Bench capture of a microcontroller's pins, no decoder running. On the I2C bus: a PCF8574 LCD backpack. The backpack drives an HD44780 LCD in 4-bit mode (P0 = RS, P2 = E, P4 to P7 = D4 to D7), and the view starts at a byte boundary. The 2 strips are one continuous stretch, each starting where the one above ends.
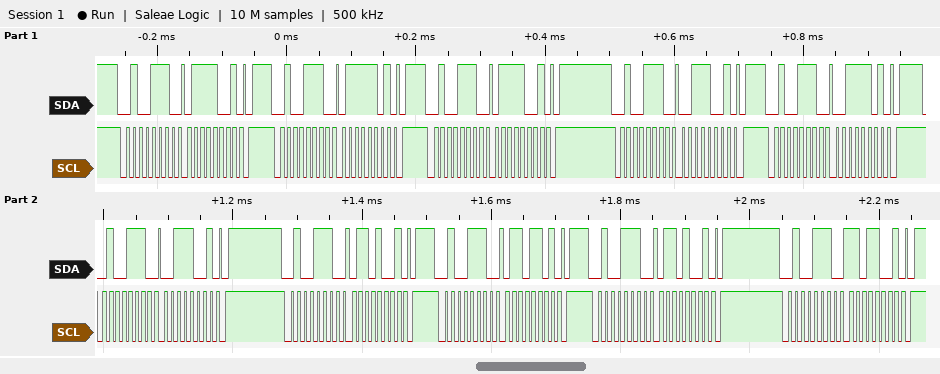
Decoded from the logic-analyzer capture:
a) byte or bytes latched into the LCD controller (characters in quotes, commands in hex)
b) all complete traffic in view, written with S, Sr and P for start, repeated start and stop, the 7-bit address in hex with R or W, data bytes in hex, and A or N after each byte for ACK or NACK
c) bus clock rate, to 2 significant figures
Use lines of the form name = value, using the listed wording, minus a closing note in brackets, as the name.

byte or bytes latched into the LCD controller = 's'
all complete traffic in view, written with S, Sr and P for start, repeated start and stop, the 7-bit address in hex with R or W, data bytes in hex, and A or N after each byte for ACK or NACK = S 27W A 79 A P S 27W A 7D A P S 27W A 79 A P S 27W A 39 A P S 27W A 3D A P S 27W A 39 A P S 27W A 69 A P S 27W A 6D A P S 27W A 69 A P S 27W A D9 A P
bus clock rate, to 2 significant figures = 100 kHz
